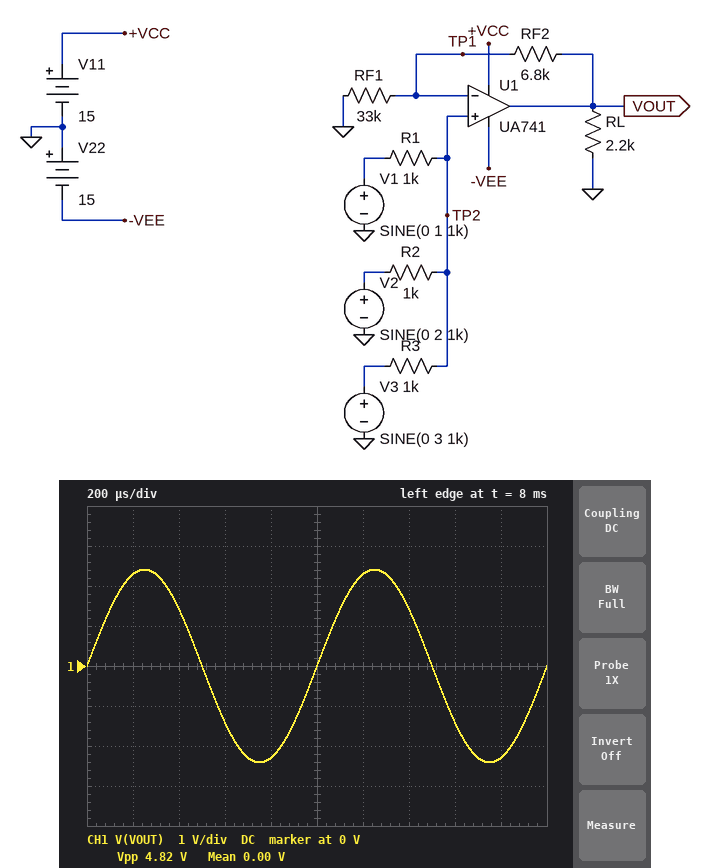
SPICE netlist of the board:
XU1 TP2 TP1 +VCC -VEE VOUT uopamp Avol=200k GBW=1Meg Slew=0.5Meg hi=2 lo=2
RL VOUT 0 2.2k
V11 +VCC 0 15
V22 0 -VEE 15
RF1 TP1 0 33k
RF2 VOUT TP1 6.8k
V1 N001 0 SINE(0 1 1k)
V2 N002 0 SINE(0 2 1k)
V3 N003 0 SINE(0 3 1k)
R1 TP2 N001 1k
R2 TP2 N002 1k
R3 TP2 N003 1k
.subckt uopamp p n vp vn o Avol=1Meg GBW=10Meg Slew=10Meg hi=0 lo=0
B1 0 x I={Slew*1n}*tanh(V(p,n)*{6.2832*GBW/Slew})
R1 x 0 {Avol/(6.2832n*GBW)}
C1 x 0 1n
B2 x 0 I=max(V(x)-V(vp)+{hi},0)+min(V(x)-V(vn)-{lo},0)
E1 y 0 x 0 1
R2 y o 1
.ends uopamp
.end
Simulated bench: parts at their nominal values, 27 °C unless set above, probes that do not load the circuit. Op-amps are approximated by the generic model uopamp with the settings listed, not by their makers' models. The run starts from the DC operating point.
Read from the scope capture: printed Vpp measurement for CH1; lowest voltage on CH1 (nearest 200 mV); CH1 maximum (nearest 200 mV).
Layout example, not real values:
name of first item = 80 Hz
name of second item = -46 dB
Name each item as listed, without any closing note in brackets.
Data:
printed Vpp measurement for CH1 = 4.82 V
lowest voltage on CH1 = -2.4 V
CH1 maximum = 2.4 V
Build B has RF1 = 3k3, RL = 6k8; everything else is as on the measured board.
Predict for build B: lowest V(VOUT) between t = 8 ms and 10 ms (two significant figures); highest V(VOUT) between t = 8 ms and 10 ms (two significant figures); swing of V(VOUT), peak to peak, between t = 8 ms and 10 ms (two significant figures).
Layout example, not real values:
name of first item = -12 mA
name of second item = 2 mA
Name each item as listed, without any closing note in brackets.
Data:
lowest V(VOUT) between t = 8 ms and 10 ms = -6.1 V
highest V(VOUT) between t = 8 ms and 10 ms = 6.1 V
swing of V(VOUT), peak to peak, between t = 8 ms and 10 ms = 12 V
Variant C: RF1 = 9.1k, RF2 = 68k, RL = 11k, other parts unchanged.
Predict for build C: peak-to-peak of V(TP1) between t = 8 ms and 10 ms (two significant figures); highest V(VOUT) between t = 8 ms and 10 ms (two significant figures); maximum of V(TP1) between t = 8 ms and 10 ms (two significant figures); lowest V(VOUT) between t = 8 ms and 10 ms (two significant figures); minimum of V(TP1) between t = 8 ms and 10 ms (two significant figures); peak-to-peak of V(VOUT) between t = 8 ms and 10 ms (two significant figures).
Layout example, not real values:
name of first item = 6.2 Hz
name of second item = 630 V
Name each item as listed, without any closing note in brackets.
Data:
peak-to-peak of V(TP1) between t = 8 ms and 10 ms = 3.1 V
highest V(VOUT) between t = 8 ms and 10 ms = 13 V
maximum of V(TP1) between t = 8 ms and 10 ms = 1.5 V
lowest V(VOUT) between t = 8 ms and 10 ms = -13 V
minimum of V(TP1) between t = 8 ms and 10 ms = -1.5 V
peak-to-peak of V(VOUT) between t = 8 ms and 10 ms = 26 V
